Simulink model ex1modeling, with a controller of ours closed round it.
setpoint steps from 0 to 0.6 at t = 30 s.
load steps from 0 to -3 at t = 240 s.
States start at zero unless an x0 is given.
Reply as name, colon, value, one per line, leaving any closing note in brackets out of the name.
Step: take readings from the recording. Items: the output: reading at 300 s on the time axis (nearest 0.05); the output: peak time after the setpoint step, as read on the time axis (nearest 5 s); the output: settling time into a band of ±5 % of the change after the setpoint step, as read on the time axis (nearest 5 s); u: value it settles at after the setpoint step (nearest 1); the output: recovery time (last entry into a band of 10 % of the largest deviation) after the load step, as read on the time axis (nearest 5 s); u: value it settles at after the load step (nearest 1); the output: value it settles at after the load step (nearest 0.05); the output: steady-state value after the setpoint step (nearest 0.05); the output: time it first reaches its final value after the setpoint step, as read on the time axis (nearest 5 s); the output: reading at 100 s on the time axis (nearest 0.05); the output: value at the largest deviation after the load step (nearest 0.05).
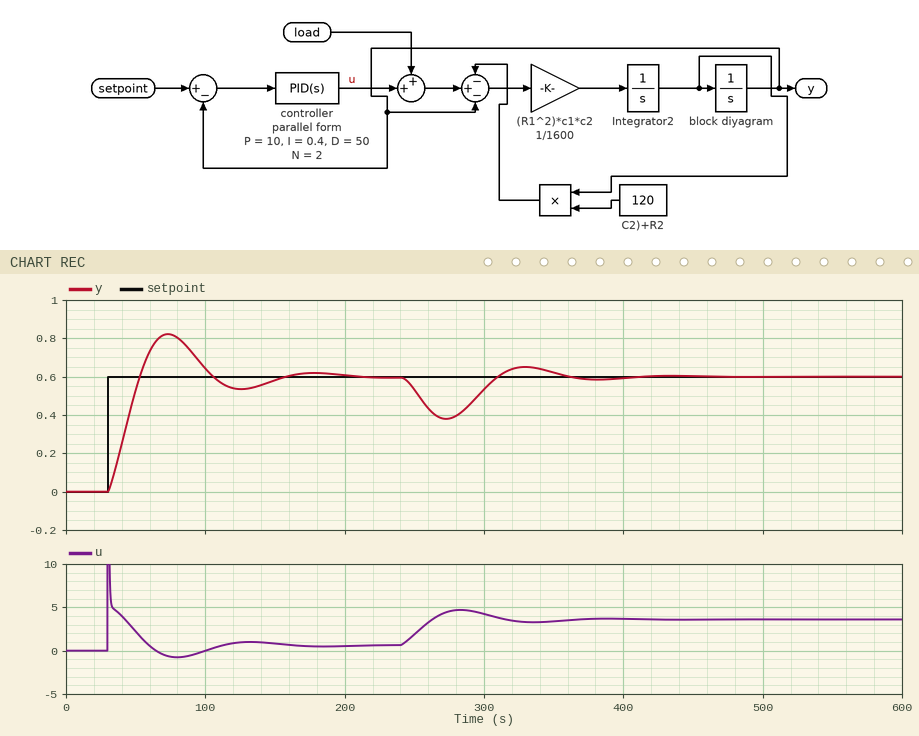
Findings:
the output: reading at 300 s on the time axis: 0.55
the output: peak time after the setpoint step, as read on the time axis: 75 s
the output: settling time into a band of ±5 % of the change after the setpoint step, as read on the time axis: 145 s
u: value it settles at after the setpoint step: 1
the output: recovery time (last entry into a band of 10 % of the largest deviation) after the load step, as read on the time axis: 350 s
u: value it settles at after the load step: 4
the output: value it settles at after the load step: 0.60
the output: steady-state value after the setpoint step: 0.60
the output: time it first reaches its final value after the setpoint step, as read on the time axis: 55 s
the output: reading at 100 s on the time axis: 0.65
the output: value at the largest deviation after the load step: 0.40
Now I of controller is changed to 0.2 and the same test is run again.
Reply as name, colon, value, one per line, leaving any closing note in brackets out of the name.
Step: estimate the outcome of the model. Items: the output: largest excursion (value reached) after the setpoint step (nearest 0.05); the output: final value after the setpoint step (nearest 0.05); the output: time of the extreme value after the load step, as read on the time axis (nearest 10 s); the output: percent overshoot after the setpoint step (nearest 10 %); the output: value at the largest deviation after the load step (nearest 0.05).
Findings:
the output: largest excursion (value reached) after the setpoint step: 0.70
the output: final value after the setpoint step: 0.60
the output: time of the extreme value after the load step, as read on the time axis: 280 s
the output: percent overshoot after the setpoint step: 20 %
the output: value at the largest deviation after the load step: 0.35
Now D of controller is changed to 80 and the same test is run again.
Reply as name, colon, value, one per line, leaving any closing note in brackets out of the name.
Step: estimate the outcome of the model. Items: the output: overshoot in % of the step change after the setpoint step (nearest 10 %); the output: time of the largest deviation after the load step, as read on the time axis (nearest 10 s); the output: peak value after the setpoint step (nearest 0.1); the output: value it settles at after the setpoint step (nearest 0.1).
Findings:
the output: overshoot in % of the step change after the setpoint step: 30 %
the output: time of the largest deviation after the load step, as read on the time axis: 270 s
the output: peak value after the setpoint step: 0.8
the output: value it settles at after the setpoint step: 0.6
